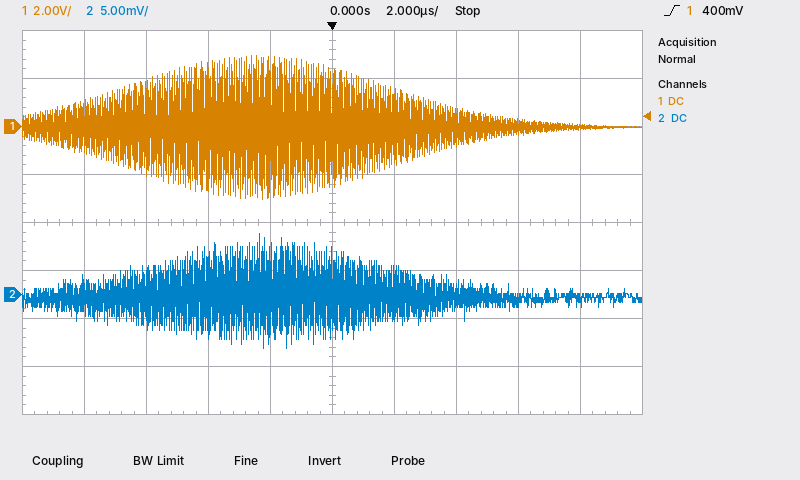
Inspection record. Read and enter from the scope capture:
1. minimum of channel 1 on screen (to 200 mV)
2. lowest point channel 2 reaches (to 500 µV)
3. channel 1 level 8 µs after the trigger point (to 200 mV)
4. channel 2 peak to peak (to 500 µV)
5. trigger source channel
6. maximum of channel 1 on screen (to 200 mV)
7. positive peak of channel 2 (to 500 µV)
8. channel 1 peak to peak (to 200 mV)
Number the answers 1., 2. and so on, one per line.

1. -3.0 V
2. -5.5 mV
3. 0.0 V
4. 12.0 mV
5. channel 1
6. 3.0 V
7. 6.5 mV
8. 6.0 V
